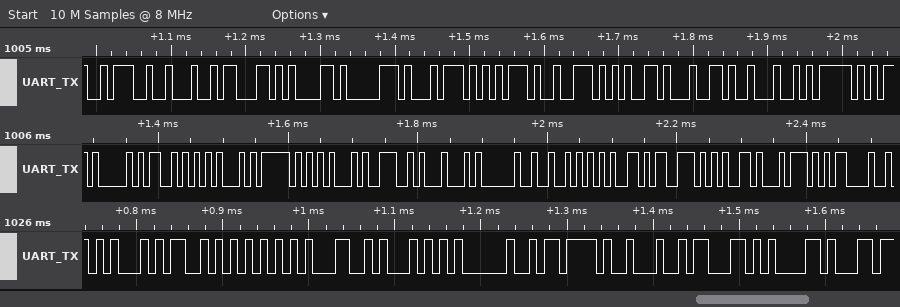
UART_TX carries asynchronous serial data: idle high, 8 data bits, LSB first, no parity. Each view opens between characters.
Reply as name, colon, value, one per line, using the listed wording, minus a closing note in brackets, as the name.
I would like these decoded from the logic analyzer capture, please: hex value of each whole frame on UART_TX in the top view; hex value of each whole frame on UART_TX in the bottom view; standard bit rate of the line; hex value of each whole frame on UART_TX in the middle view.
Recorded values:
hex value of each whole frame on UART_TX in the top view: 3A, 22, 63, 61, 70, 74, 75, 72, 65, 64, 22, 7D
hex value of each whole frame on UART_TX in the bottom view: 45, 53, 55, 4C, 54, 20, 7B, 22, 63, 61
standard bit rate of the line: 115200 baud
hex value of each whole frame on UART_TX in the middle view: 41, 53, 45, 5F, 45, 4E, 44, 20, 52, 65, 73, 65, 74, 0D
